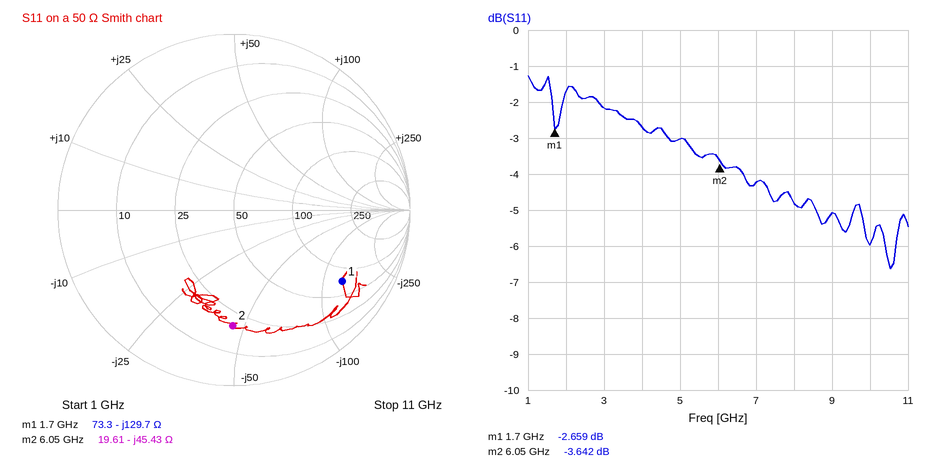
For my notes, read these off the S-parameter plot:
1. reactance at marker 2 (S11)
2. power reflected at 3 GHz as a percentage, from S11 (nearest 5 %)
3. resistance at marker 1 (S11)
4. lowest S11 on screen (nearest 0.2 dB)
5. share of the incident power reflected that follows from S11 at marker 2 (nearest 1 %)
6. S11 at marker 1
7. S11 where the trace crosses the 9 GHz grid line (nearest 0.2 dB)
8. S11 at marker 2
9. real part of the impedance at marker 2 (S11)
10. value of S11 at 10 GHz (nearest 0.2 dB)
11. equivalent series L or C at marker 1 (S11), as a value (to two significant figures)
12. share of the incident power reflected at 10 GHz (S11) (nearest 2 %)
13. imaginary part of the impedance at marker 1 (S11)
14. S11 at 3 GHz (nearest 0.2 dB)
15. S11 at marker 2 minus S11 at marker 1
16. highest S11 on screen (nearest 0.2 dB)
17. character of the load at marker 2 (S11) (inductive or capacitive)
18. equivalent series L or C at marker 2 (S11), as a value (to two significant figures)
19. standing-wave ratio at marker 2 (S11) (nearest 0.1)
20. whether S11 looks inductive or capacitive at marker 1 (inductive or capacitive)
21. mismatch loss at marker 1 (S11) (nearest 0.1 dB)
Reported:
-45.43 Ω
60 %
73.3 Ω
-6.6 dB
43 %
-2.659 dB
-5.0 dB
-3.642 dB
19.61 Ω
-6.0 dB
720 fF
26 %
-129.7 Ω
-2.2 dB
-0.983 dB
-1.2 dB
capacitive
580 fF
4.8
capacitive
3.4 dB
